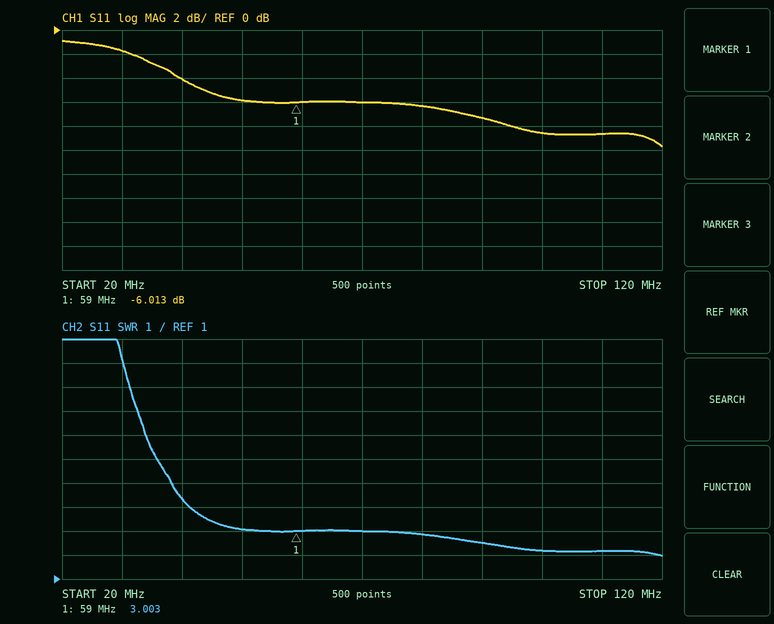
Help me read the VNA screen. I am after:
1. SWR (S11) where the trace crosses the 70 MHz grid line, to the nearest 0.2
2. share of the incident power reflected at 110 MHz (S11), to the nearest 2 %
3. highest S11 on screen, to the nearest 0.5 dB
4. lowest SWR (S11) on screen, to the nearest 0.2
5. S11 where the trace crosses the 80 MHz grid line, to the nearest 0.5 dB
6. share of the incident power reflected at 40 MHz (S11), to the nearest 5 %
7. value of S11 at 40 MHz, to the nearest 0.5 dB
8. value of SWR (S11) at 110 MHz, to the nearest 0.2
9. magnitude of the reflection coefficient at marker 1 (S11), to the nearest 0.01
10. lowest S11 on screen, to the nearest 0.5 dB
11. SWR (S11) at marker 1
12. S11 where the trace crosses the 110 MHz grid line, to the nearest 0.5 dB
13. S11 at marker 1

3.0
14 %
-1.0 dB
2.0
-6.5 dB
40 %
-4.0 dB
2.2
0.50
-9.5 dB
3.003
-8.5 dB
-6.013 dB
